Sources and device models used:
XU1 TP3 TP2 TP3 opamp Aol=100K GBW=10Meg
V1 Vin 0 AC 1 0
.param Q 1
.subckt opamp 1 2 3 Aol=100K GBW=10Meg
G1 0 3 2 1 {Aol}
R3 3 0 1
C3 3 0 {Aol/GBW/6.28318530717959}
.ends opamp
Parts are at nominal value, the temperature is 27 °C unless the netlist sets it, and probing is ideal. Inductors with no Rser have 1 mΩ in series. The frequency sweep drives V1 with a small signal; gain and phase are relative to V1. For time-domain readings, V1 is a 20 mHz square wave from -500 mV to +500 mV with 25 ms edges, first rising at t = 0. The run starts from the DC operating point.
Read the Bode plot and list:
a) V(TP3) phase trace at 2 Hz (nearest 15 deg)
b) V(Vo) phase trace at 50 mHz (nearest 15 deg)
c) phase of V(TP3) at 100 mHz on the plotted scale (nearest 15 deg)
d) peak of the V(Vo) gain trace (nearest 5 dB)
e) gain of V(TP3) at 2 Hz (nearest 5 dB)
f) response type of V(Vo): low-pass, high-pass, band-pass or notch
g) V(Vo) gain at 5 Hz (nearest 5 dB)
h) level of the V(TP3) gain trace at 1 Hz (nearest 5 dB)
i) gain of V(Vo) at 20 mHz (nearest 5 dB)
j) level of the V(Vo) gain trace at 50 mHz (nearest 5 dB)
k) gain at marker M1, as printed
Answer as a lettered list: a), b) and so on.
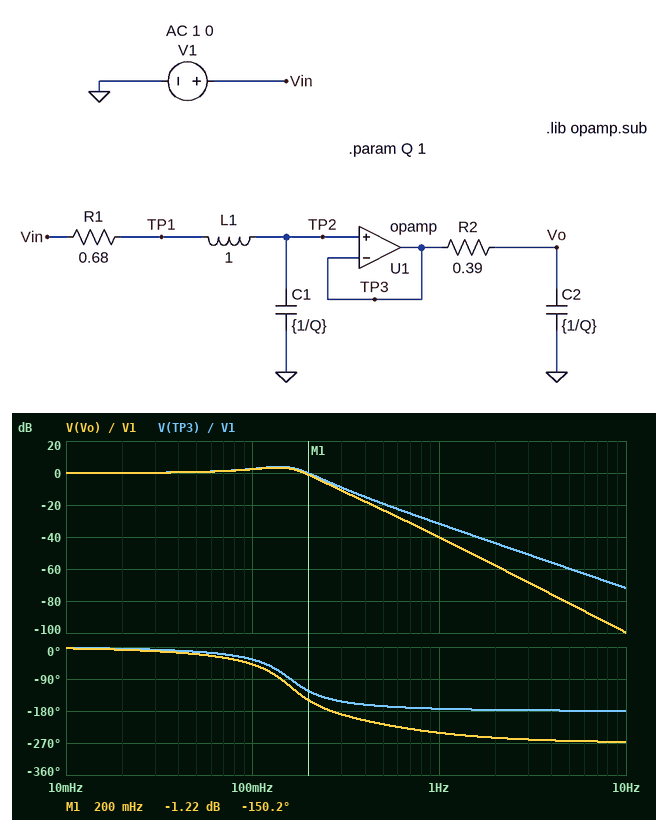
a) -180 deg
b) -15 deg
c) -30 deg
d) 5 dB
e) -45 dB
f) low-pass
g) -80 dB
h) -30 dB
i) 0 dB
j) 0 dB
k) -1.22 dB
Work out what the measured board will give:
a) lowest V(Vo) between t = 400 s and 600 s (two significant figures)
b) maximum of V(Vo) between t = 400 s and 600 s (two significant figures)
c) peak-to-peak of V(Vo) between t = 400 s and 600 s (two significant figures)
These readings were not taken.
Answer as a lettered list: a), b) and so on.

a) -800 mV
b) 800 mV
c) 1.6 V
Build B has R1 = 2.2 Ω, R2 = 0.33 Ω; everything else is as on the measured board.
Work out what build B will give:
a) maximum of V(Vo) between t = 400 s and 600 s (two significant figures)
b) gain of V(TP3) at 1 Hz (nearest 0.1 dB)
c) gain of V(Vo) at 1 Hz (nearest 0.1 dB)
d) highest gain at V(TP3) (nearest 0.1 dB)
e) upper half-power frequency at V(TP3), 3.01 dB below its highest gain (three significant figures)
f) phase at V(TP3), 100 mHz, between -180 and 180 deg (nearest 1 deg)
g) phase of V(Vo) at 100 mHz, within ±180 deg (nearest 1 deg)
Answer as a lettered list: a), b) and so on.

a) 500 mV
b) -32.2 dB
c) -39.5 dB
d) 0 dB
e) 89.5 mHz
f) -66 deg
g) -78 deg
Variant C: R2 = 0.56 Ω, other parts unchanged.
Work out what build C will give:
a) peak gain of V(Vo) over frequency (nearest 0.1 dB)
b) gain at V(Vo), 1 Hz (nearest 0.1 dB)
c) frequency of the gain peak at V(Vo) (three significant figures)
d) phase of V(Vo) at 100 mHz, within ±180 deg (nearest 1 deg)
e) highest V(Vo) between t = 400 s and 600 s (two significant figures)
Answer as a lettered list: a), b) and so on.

a) 3.0 dB
b) -43.0 dB
c) 135 mHz
d) -55 deg
e) 770 mV
